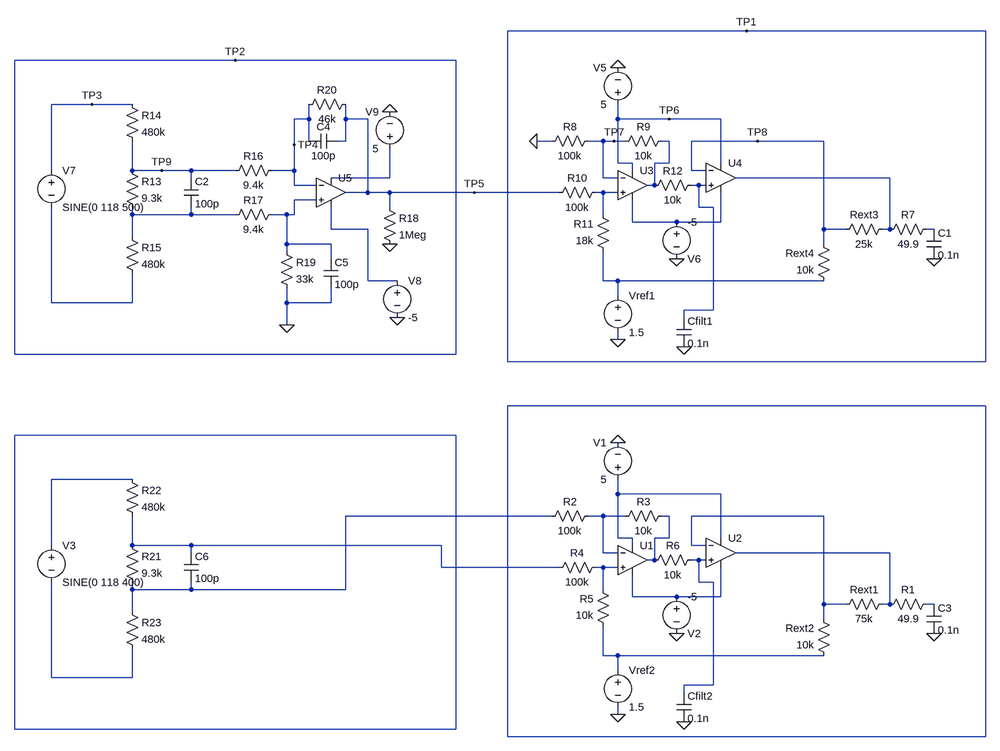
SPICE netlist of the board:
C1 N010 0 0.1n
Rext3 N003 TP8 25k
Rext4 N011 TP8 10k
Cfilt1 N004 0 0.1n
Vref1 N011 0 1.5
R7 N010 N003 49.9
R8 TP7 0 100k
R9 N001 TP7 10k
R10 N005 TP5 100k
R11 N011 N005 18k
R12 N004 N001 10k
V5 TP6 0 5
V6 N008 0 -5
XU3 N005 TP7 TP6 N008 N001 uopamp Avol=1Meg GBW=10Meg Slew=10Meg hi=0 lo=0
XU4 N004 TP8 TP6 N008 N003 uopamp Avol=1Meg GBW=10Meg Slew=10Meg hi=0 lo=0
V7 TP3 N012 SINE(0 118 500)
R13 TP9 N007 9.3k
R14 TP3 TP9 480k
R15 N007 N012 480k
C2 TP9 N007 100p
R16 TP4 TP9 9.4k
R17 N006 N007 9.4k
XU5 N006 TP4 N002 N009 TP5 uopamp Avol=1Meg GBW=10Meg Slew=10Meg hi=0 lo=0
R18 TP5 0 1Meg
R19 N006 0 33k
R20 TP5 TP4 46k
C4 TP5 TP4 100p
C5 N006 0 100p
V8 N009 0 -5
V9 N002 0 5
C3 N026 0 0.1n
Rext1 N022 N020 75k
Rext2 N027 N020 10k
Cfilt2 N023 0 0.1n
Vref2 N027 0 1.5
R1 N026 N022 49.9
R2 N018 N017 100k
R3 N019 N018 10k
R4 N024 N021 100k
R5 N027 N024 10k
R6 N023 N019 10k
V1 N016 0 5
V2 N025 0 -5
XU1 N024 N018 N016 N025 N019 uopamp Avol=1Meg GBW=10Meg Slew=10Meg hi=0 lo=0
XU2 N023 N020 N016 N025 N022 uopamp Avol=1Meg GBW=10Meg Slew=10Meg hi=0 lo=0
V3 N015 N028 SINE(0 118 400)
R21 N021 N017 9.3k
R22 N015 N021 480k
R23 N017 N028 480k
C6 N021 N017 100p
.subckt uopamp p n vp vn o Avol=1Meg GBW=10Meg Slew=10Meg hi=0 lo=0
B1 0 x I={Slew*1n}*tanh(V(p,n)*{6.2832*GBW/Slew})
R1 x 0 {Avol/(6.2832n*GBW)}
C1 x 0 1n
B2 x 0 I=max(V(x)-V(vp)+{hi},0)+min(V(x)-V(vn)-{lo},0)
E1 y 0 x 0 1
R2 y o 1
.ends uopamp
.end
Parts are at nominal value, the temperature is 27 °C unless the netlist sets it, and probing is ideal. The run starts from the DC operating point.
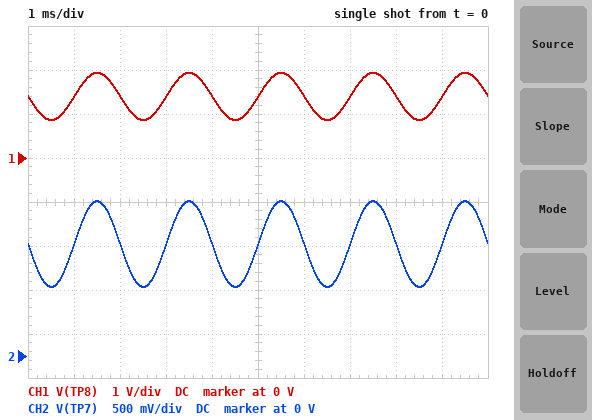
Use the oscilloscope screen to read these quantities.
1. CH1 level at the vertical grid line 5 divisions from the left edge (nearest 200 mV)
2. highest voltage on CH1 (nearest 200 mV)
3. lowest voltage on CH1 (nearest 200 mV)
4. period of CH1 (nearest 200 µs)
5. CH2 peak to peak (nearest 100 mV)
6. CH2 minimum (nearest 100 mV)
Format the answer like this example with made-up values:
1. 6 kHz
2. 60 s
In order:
1. 1.4 V
2. 2.0 V
3. 800 mV
4. 2.0 ms
5. 1.0 V
6. 800 mV
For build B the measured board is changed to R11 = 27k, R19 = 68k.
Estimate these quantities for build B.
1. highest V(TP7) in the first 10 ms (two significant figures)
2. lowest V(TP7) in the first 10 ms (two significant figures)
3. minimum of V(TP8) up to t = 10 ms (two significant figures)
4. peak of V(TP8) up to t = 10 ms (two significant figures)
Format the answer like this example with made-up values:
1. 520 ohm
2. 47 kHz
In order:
1. 2.2 V
2. 200 mV
3. 220 mV
4. 2.4 V
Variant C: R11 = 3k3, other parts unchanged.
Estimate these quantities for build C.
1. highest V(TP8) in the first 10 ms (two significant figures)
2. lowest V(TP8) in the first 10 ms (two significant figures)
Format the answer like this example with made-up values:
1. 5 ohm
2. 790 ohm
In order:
1. 1.7 V
2. 1.5 V
